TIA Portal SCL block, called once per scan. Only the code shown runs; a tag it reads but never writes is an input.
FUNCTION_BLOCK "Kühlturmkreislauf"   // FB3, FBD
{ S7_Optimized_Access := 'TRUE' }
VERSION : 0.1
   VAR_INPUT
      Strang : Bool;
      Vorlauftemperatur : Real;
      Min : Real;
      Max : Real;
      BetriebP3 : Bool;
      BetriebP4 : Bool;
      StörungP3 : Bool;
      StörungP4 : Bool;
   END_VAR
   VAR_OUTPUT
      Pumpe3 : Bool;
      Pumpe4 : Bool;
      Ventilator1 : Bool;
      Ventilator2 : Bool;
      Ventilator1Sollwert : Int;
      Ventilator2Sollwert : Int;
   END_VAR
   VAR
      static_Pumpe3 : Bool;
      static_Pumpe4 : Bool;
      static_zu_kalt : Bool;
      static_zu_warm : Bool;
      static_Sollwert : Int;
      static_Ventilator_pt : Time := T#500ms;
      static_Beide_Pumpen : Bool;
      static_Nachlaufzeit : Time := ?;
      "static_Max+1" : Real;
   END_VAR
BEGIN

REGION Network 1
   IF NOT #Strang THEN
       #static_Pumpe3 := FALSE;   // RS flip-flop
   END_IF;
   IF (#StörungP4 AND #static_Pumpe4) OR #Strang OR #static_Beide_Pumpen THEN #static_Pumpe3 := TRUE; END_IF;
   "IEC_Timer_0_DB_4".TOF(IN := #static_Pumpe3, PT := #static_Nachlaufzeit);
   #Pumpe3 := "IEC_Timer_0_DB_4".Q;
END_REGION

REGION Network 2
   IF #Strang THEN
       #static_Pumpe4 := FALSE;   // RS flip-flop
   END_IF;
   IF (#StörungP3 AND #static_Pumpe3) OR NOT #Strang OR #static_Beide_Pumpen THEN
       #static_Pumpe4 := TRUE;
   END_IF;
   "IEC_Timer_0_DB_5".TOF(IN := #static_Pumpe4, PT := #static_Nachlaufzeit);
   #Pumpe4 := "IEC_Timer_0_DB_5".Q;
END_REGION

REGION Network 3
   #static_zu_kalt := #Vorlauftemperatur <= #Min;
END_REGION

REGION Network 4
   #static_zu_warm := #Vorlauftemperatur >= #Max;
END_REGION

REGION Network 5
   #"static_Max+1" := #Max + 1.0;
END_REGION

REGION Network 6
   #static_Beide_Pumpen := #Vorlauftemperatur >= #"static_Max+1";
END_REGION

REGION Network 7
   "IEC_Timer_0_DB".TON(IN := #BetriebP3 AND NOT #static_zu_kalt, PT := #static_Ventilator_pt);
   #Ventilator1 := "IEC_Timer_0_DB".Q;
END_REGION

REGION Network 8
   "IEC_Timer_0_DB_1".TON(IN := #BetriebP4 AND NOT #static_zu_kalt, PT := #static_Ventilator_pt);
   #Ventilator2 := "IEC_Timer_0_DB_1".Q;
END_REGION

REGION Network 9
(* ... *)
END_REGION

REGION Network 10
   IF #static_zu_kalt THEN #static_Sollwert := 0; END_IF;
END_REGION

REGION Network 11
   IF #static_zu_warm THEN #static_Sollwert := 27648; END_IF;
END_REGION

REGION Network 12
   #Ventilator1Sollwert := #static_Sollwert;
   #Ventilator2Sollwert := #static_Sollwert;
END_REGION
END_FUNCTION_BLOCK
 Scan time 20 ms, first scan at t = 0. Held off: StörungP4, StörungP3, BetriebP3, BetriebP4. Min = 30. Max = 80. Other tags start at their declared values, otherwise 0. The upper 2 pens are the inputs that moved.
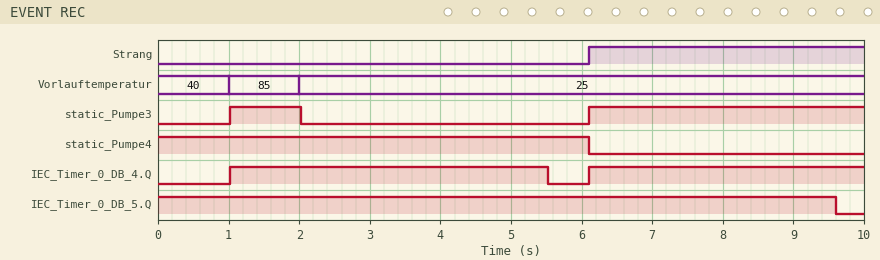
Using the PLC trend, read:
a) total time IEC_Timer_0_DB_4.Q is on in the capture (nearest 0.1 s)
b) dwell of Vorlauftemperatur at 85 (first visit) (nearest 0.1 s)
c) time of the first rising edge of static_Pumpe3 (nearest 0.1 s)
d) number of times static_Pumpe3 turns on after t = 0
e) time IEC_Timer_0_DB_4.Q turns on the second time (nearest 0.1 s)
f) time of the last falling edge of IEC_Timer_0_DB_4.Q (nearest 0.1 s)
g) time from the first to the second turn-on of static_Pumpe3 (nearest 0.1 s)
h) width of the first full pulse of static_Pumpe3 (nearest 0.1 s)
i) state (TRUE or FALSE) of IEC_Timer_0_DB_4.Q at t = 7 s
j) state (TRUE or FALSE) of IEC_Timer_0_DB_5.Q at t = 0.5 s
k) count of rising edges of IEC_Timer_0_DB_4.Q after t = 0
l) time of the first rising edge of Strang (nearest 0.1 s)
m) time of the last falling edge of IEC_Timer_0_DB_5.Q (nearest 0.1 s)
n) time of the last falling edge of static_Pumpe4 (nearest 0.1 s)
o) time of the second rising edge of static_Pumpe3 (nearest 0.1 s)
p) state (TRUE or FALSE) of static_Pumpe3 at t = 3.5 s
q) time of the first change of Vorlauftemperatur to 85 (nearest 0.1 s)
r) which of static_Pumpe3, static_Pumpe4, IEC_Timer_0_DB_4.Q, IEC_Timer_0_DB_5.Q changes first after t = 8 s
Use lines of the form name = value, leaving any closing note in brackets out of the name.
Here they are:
total time IEC_Timer_0_DB_4.Q is on in the capture = 8.4 s
dwell of Vorlauftemperatur at 85 (first visit) = 1.0 s
time of the first rising edge of static_Pumpe3 = 1.0 s
number of times static_Pumpe3 turns on after t = 0 = 2
time IEC_Timer_0_DB_4.Q turns on the second time = 6.1 s
time of the last falling edge of IEC_Timer_0_DB_4.Q = 5.5 s
time from the first to the second turn-on of static_Pumpe3 = 5.1 s
width of the first full pulse of static_Pumpe3 = 1.0 s
state (TRUE or FALSE) of IEC_Timer_0_DB_4.Q at t = 7 s = TRUE
state (TRUE or FALSE) of IEC_Timer_0_DB_5.Q at t = 0.5 s = TRUE
count of rising edges of IEC_Timer_0_DB_4.Q after t = 0 = 2
time of the first rising edge of Strang = 6.1 s
time of the last falling edge of IEC_Timer_0_DB_5.Q = 9.6 s
time of the last falling edge of static_Pumpe4 = 6.1 s
time of the second rising edge of static_Pumpe3 = 6.1 s
state (TRUE or FALSE) of static_Pumpe3 at t = 3.5 s = FALSE
time of the first change of Vorlauftemperatur to 85 = 1.0 s
which of static_Pumpe3, static_Pumpe4, IEC_Timer_0_DB_4.Q, IEC_Timer_0_DB_5.Q changes first after t = 8 s = IEC_Timer_0_DB_5.Q
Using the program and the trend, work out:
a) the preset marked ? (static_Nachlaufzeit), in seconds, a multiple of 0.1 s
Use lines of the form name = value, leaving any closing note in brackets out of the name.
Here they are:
the preset marked ? (static_Nachlaufzeit), in seconds, a multiple of 0.1 s = 3.5 s
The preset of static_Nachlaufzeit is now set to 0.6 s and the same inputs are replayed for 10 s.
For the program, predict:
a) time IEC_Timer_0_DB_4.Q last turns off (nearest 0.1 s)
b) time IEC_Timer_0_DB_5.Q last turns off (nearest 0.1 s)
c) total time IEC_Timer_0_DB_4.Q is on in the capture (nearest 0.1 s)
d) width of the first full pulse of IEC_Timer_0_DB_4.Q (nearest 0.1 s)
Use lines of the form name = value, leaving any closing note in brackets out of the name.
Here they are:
time IEC_Timer_0_DB_4.Q last turns off = 2.6 s
time IEC_Timer_0_DB_5.Q last turns off = 6.7 s
total time IEC_Timer_0_DB_4.Q is on in the capture = 5.5 s
width of the first full pulse of IEC_Timer_0_DB_4.Q = 1.6 s
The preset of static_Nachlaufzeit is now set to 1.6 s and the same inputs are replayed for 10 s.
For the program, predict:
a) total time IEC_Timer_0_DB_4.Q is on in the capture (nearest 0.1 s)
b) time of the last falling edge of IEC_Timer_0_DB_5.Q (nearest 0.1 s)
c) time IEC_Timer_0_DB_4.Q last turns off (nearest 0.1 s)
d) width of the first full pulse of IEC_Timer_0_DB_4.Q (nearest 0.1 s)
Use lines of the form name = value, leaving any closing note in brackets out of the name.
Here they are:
total time IEC_Timer_0_DB_4.Q is on in the capture = 6.5 s
time of the last falling edge of IEC_Timer_0_DB_5.Q = 7.7 s
time IEC_Timer_0_DB_4.Q last turns off = 3.6 s
width of the first full pulse of IEC_Timer_0_DB_4.Q = 2.6 s
